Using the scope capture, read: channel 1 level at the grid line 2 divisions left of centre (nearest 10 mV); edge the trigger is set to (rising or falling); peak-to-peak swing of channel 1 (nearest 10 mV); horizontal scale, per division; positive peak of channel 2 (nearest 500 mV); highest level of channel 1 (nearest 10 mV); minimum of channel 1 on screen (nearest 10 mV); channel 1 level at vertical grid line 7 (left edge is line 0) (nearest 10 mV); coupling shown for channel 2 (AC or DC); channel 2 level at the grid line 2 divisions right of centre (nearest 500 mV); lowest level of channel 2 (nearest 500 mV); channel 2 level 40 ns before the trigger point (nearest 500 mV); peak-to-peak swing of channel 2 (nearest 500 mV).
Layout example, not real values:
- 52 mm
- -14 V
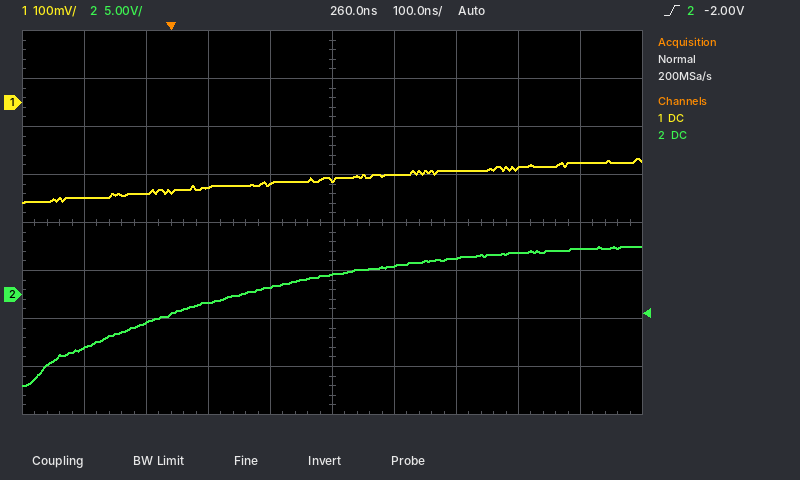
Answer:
- -180 mV
- rising
- 90 mV
- 100 ns
- 5.0 V
- -120 mV
- -210 mV
- -140 mV
- DC
- 4.0 V
- -9.5 V
- -3.0 V
- 14.5 V
